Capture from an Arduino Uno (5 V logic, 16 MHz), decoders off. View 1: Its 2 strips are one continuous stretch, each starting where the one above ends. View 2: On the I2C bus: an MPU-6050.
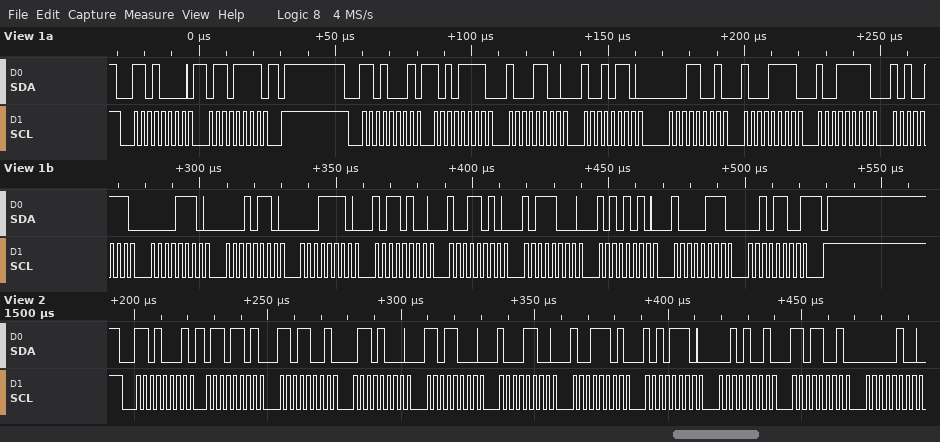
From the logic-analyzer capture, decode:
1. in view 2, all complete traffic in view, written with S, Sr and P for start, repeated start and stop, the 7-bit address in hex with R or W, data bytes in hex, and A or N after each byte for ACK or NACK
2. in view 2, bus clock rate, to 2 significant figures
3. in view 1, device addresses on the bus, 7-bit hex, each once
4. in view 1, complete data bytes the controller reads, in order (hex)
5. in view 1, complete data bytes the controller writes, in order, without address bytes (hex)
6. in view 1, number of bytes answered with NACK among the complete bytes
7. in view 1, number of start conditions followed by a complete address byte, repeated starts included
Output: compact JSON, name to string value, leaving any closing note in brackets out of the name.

{"in view 2, all complete traffic in view, written with S, Sr and P for start, repeated start and stop, the 7-bit address in hex with R or W, data bytes in hex, and A or N after each byte for ACK or NACK": "S 68R A 6D A D9 A 68 A D8 A 8C A 9D A AE A 29 A D9 A 04 A", "in view 2, bus clock rate, to 2 significant figures": "400 kHz", "in view 1, device addresses on the bus, 7-bit hex, each once": "0x68", "in view 1, complete data bytes the controller reads, in order": "AF 8C 96 19 8F 9F A7 0E 16 1E B4 9A B8 AA 87 2C", "in view 1, complete data bytes the controller writes, in order, without address bytes": "6F", "in view 1, number of bytes answered with NACK among the complete bytes": "1", "in view 1, number of start conditions followed by a complete address byte, repeated starts included": "2"}
